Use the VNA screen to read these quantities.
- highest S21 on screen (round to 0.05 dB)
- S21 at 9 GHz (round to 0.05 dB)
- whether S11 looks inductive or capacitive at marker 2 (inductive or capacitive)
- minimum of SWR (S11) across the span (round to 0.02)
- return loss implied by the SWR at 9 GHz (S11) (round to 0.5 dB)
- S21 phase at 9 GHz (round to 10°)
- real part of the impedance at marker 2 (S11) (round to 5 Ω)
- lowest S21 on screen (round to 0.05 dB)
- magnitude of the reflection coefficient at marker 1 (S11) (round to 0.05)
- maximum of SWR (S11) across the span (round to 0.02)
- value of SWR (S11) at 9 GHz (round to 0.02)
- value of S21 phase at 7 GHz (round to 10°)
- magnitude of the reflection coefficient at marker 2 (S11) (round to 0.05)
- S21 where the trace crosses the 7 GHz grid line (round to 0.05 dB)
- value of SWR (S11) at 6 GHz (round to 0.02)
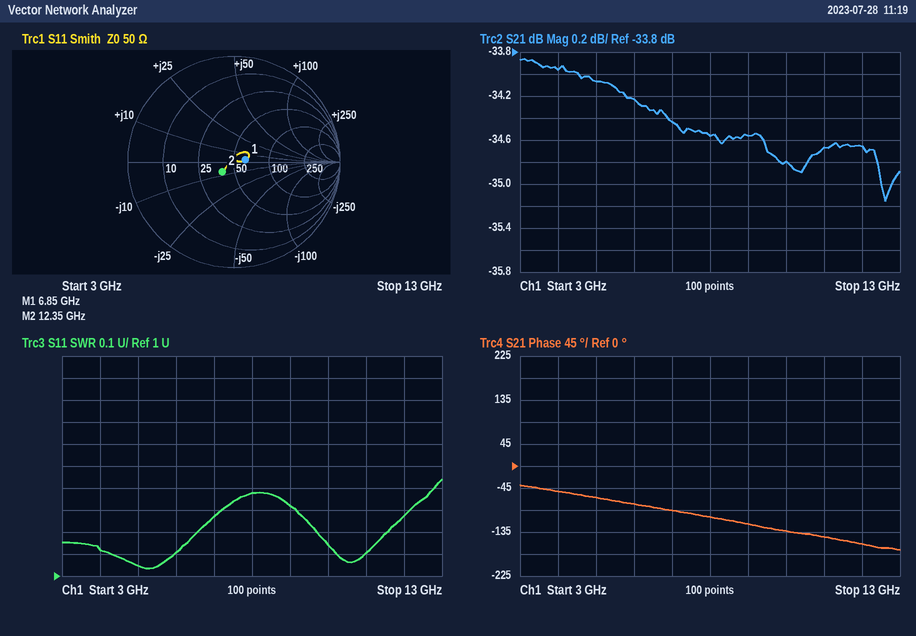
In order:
-33.85 dB
-34.55 dB
capacitive
1.04
17.0 dB
-120°
40 Ω
-35.15 dB
0.10
1.44
1.32
-90°
0.15
-34.45 dB
1.10
